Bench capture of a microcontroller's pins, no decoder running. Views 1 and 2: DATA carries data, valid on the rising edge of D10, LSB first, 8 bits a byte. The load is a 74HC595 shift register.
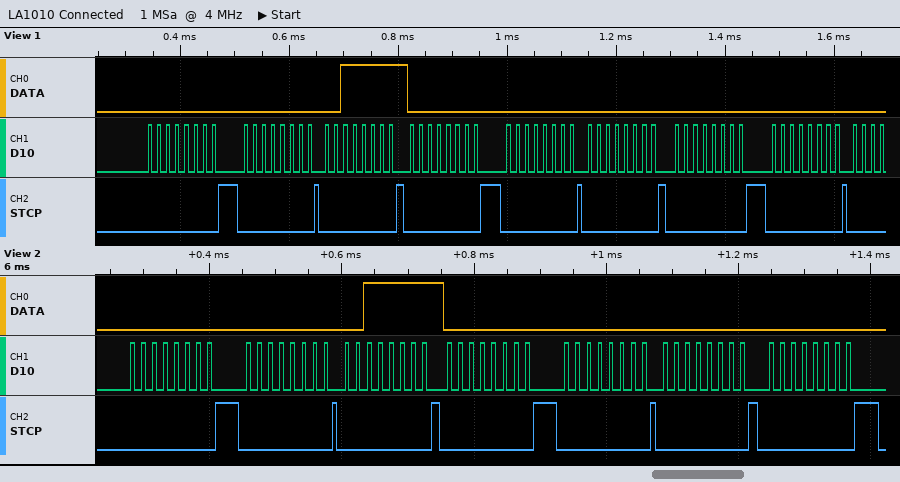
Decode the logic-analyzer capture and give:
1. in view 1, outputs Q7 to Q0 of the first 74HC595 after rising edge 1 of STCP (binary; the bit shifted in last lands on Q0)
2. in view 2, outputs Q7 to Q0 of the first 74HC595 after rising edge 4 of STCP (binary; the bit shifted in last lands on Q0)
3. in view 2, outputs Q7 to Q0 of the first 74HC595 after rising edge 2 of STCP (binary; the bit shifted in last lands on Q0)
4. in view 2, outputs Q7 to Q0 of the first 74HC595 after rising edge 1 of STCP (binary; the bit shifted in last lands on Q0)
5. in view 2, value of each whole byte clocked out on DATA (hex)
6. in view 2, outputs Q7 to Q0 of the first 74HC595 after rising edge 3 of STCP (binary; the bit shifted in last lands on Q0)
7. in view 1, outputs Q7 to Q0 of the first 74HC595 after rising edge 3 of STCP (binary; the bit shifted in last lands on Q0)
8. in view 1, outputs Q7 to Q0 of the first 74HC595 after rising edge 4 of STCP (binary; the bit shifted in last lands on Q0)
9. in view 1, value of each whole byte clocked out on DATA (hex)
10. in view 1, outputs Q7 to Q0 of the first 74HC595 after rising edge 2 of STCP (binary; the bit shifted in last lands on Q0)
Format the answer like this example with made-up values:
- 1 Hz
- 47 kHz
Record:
- 00000000
- 00000000
- 00000000
- 00000000
- 0x00 0x00 0xFC 0x00 0x00 0x00 0x00
- 00111111
- 00111111
- 00000000
- 00 00 FC 00 00 00 00 00
- 00000000
